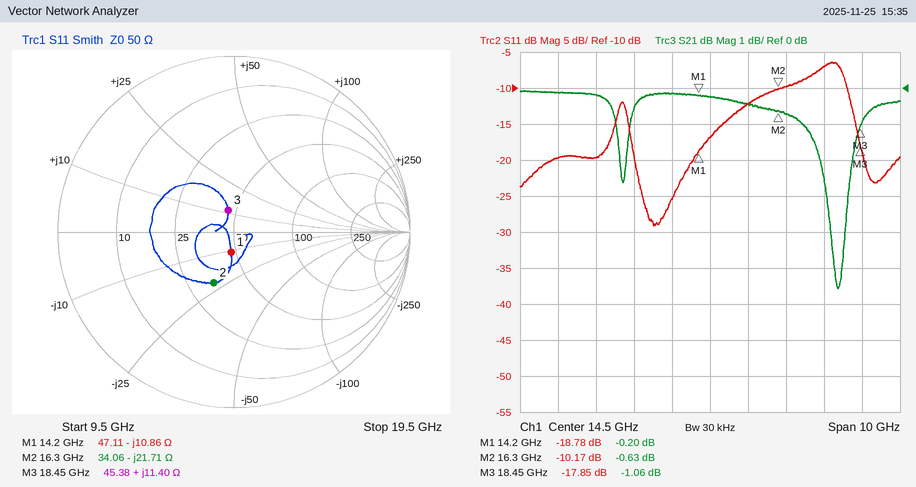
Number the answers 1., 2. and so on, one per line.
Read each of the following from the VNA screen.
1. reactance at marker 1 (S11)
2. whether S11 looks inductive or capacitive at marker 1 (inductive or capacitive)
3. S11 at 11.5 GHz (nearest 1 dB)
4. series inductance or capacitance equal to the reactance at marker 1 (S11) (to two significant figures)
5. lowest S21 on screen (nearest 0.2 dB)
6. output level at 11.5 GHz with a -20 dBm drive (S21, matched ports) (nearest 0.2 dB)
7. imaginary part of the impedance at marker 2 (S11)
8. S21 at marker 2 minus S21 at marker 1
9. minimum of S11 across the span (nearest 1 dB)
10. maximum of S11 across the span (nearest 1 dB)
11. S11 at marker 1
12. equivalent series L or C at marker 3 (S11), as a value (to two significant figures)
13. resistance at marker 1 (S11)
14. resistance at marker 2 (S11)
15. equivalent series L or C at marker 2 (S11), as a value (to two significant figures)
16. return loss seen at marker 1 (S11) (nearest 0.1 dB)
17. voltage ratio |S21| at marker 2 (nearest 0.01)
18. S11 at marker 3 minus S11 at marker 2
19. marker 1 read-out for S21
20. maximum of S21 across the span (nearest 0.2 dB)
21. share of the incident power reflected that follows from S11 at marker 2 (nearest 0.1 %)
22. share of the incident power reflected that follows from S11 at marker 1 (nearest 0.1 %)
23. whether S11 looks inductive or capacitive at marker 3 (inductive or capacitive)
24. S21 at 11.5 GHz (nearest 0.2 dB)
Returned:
1. -10.86 Ω
2. capacitive
3. -20 dB
4. 1.0 pF
5. -5.6 dB
6. -20.2 dBm
7. -21.71 Ω
8. -0.43 dB
9. -29 dB
10. -6 dB
11. -18.78 dB
12. 98 pH
13. 47.11 Ω
14. 34.06 Ω
15. 450 fF
16. 18.8 dB
17. 0.93
18. -7.68 dB
19. -0.20 dB
20. 0.0 dB
21. 9.6 %
22. 1.3 %
23. inductive
24. -0.2 dB
